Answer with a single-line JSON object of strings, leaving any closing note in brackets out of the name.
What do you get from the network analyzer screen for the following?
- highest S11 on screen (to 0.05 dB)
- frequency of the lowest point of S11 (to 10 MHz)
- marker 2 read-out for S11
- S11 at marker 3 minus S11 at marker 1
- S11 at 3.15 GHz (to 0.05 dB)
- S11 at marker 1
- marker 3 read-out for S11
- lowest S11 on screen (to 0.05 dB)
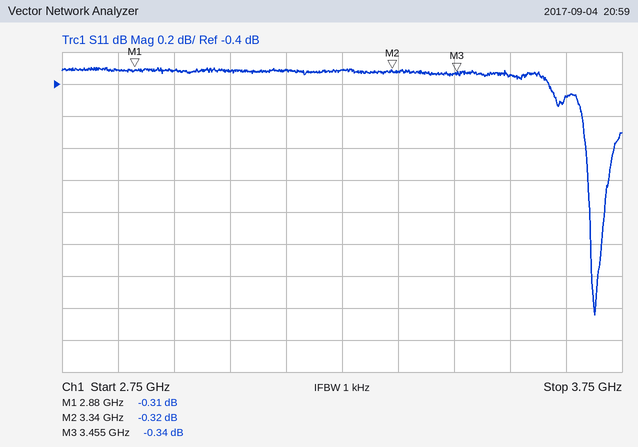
{"highest S11 on screen": "-0.30 dB", "frequency of the lowest point of S11": "3.70 GHz", "marker 2 read-out for S11": "-0.32 dB", "S11 at marker 3 minus S11 at marker 1": "-0.03 dB", "S11 at 3.15 GHz": "-0.30 dB", "S11 at marker 1": "-0.31 dB", "marker 3 read-out for S11": "-0.34 dB", "lowest S11 on screen": "-1.85 dB"}
